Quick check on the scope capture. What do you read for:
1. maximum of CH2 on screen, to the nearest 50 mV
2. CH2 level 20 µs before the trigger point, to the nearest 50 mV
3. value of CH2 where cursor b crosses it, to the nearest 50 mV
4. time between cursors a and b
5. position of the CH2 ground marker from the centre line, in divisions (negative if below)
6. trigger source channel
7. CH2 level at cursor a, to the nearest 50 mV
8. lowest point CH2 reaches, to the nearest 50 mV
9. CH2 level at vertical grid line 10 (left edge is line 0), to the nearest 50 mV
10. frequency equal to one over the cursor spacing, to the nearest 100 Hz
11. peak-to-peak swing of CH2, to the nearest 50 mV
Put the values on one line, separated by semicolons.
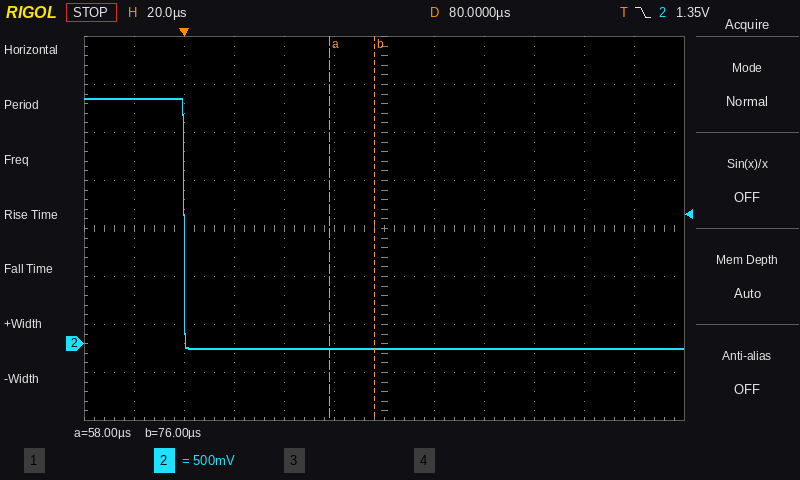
2.55 V; 2.55 V; -50 mV; 18 µs; -2.4 div; CH2; -50 mV; -50 mV; -50 mV; 55.6 kHz; 2.60 V
